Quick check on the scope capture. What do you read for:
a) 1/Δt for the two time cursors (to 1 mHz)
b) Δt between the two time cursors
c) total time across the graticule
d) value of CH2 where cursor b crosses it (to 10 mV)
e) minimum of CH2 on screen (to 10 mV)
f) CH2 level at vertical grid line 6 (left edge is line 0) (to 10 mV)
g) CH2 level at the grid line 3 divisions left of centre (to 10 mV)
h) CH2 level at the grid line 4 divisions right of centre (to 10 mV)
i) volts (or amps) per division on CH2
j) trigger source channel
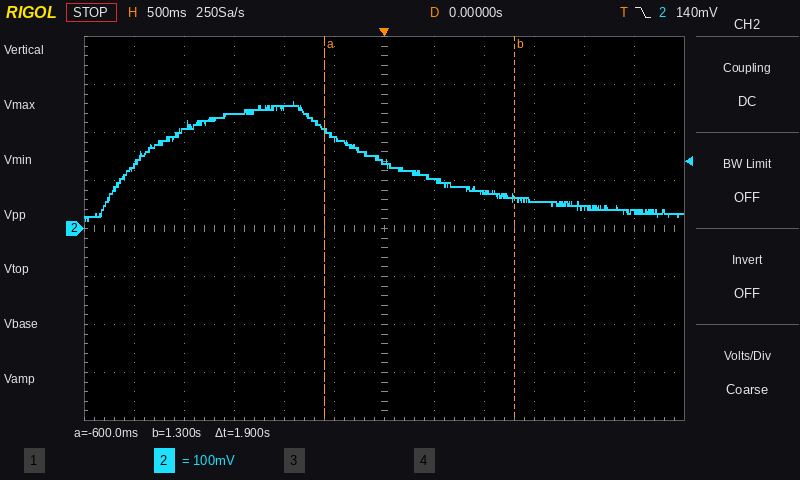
526 mHz
1.9 s
6 s
60 mV
20 mV
140 mV
240 mV
40 mV
100 mV
CH2
